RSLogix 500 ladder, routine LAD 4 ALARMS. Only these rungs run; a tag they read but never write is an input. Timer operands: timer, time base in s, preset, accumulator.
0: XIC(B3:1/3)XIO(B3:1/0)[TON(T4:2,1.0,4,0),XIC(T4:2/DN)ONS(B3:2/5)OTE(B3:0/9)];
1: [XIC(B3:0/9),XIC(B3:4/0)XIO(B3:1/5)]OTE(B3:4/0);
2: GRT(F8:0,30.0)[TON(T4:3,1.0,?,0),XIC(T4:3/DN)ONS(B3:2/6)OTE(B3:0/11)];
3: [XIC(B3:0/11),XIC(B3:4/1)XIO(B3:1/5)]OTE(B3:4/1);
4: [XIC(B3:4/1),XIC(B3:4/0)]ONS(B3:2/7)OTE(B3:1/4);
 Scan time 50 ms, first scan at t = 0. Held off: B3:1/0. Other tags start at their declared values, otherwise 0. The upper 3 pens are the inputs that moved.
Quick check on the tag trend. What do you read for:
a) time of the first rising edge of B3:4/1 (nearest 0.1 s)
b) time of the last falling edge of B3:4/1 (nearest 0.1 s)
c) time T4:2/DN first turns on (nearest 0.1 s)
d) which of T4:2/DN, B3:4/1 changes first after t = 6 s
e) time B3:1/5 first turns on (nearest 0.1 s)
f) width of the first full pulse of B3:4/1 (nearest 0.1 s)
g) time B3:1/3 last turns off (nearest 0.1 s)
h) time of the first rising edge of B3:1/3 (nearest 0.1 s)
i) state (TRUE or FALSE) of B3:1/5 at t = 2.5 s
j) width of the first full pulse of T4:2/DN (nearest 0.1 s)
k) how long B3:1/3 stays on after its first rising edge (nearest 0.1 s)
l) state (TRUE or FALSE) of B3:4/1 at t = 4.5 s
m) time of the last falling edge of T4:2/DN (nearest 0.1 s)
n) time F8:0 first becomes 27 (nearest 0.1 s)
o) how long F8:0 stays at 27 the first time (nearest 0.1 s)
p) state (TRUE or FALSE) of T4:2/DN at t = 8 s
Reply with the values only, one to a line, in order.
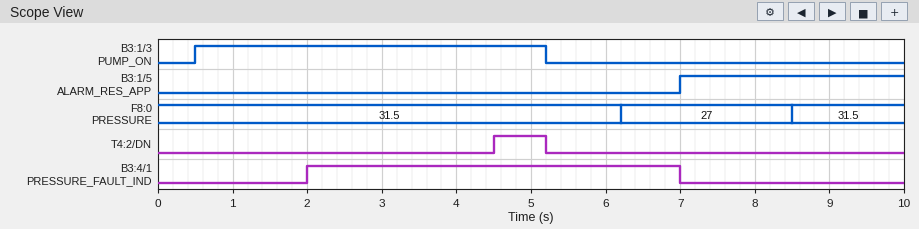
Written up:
2.0 s
7.0 s
4.5 s
B3:4/1
7.0 s
5.0 s
5.2 s
0.5 s
FALSE
0.7 s
4.7 s
TRUE
5.2 s
6.2 s
2.3 s
FALSE
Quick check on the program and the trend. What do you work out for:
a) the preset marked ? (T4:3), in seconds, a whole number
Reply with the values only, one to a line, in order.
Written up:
2 s
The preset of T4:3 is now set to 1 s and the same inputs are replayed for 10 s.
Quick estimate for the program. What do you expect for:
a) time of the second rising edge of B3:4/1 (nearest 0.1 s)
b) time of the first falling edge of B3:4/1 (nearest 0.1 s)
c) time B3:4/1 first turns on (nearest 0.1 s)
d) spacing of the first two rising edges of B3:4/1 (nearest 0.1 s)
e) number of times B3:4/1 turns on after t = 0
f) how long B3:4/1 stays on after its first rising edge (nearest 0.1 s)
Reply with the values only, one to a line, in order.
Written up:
9.5 s
7.0 s
1.0 s
8.5 s
2
6.0 s
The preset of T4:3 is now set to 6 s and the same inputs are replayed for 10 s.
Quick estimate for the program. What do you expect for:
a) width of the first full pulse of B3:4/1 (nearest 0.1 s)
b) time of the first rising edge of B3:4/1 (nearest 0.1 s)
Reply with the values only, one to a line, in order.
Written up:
1.0 s
6.0 s
